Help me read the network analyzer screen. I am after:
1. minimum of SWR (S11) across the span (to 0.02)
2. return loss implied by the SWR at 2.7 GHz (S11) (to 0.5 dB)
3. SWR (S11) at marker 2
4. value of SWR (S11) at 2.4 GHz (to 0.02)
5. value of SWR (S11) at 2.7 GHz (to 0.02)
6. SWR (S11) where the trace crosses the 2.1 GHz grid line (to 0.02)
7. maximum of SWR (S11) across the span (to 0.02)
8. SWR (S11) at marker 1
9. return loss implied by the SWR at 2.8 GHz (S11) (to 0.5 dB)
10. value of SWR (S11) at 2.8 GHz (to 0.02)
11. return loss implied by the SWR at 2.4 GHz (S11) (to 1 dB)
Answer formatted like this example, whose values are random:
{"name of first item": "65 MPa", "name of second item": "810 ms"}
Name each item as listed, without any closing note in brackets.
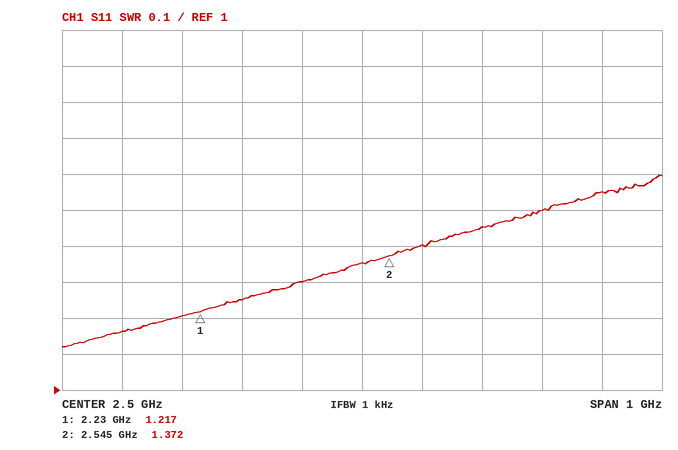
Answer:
{"minimum of SWR (S11) across the span": "1.12", "return loss implied by the SWR at 2.7 GHz (S11)": "14.5 dB", "SWR (S11) at marker 2": "1.372", "value of SWR (S11) at 2.4 GHz": "1.30", "value of SWR (S11) at 2.7 GHz": "1.46", "SWR (S11) where the trace crosses the 2.1 GHz grid line": "1.16", "maximum of SWR (S11) across the span": "1.60", "SWR (S11) at marker 1": "1.217", "return loss implied by the SWR at 2.8 GHz (S11)": "14.0 dB", "value of SWR (S11) at 2.8 GHz": "1.50", "return loss implied by the SWR at 2.4 GHz (S11)": "18 dB"}
